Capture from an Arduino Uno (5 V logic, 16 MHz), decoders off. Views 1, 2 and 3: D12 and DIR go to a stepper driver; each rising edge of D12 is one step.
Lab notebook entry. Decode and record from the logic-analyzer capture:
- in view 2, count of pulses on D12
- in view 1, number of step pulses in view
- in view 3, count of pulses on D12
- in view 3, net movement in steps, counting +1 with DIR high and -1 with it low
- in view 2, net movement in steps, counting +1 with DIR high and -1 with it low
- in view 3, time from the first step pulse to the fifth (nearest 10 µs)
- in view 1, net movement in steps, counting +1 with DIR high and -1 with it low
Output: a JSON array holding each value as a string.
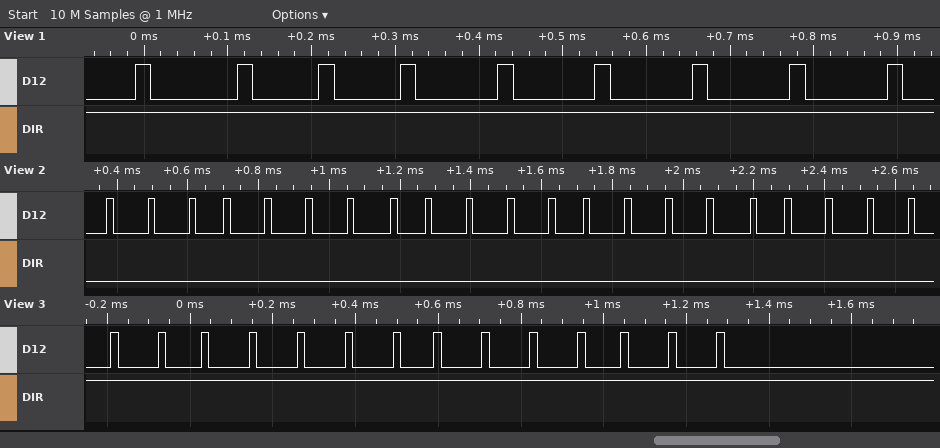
["21", "9", "14", "+14", "-21", "450 µs", "+9"]
